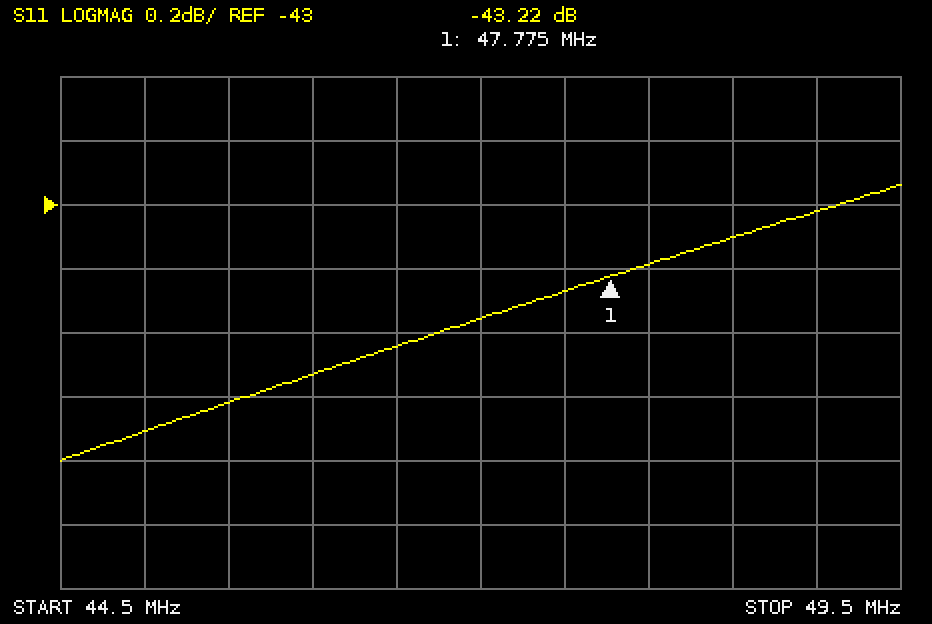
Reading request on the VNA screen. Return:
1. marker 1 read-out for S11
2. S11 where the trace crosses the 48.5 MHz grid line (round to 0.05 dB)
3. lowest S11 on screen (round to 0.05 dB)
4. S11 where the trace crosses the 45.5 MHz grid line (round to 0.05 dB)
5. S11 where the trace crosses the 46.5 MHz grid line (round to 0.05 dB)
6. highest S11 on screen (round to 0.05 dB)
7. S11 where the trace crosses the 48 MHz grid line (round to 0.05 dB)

-43.22 dB
-43.10 dB
-43.80 dB
-43.60 dB
-43.45 dB
-42.95 dB
-43.20 dB
